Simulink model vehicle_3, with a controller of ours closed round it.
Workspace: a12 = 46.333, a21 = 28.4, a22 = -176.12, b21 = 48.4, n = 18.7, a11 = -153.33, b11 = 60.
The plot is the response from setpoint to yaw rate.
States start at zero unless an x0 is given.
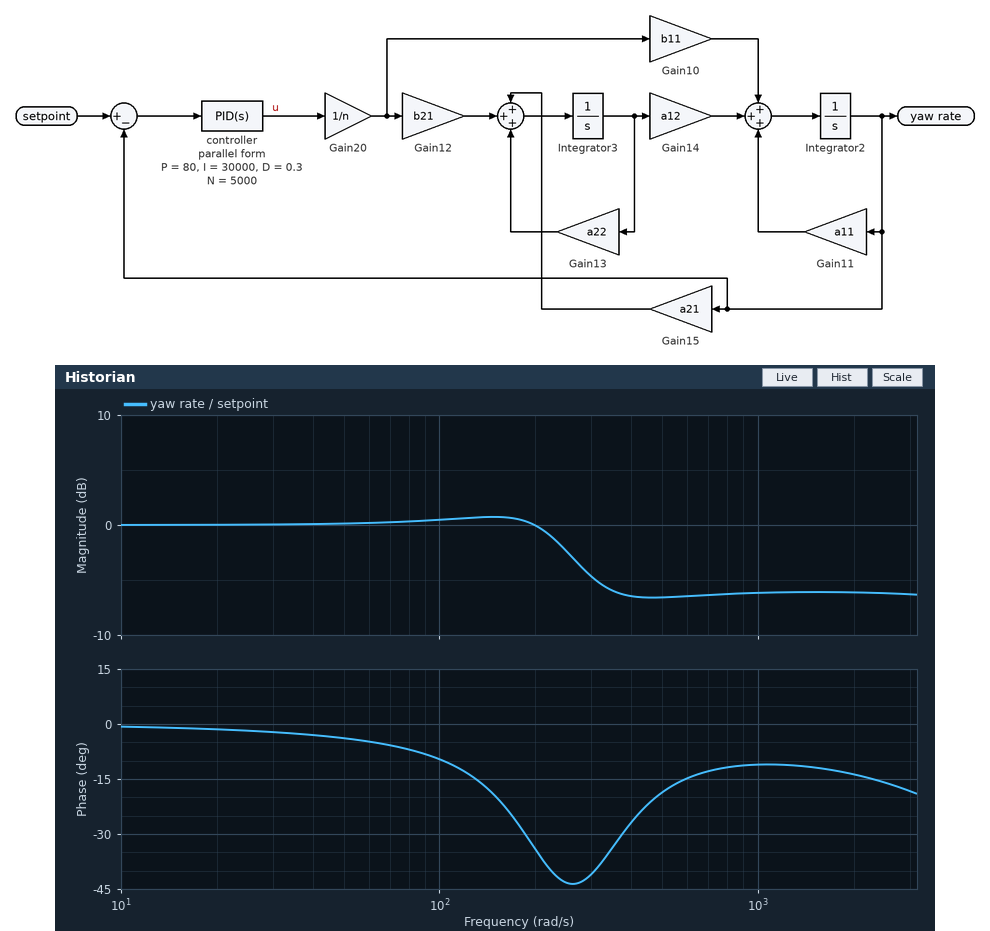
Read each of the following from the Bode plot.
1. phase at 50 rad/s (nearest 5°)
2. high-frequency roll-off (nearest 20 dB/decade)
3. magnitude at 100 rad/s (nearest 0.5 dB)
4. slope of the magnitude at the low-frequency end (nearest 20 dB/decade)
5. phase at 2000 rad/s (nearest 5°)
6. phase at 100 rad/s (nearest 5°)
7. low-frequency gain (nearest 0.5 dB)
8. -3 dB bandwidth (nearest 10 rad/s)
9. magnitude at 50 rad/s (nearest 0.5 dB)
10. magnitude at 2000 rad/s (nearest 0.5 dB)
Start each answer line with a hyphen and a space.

- -5°
- 0 dB/decade
- 0.5 dB
- 0 dB/decade
- -15°
- -10°
- 0.0 dB
- 260 rad/s
- 0.0 dB
- -6.0 dB
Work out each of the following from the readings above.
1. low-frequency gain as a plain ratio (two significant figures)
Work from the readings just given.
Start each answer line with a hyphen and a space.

- 1.0
